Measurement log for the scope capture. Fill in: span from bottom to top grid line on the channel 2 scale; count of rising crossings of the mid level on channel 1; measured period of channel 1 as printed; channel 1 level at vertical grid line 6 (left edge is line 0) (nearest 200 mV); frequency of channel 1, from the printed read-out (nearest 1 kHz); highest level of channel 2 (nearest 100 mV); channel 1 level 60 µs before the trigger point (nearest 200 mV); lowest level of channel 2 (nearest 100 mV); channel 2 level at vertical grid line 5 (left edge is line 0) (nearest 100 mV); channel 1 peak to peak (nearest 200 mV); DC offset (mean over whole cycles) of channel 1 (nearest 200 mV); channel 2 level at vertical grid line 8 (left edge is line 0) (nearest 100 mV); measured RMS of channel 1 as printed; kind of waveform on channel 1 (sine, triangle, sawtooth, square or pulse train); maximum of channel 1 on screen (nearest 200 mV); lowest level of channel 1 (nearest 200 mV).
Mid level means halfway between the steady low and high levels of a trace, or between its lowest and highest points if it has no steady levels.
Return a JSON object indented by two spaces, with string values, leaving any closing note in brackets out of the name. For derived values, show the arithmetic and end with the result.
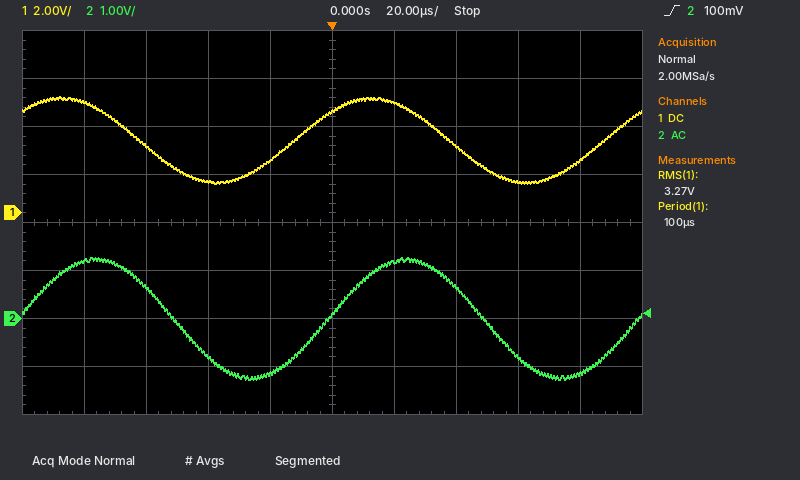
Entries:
{
  "span from bottom to top grid line on the channel 2 scale": "8 V",
  "count of rising crossings of the mid level on channel 1": "2",
  "measured period of channel 1 as printed": "100 µs",
  "channel 1 level at vertical grid line 6 (left edge is line 0)": "4.6 V",
  "frequency of channel 1, from the printed read-out": "1 / 100 µs ≈ 10 kHz",
  "highest level of channel 2": "1.3 V",
  "channel 1 level 60 µs before the trigger point": "2.8 V",
  "lowest level of channel 2": "-1.3 V",
  "channel 2 level at vertical grid line 5 (left edge is line 0)": "100 mV",
  "channel 1 peak to peak": "4.8 V − (1.2 V) = 3.6 V",
  "DC offset (mean over whole cycles) of channel 1": "(4.8 V + (1.2 V)) / 2 ≈ 3.0 V",
  "channel 2 level at vertical grid line 8 (left edge is line 0)": "-800 mV",
  "measured RMS of channel 1 as printed": "3.27 V",
  "kind of waveform on channel 1": "sine",
  "maximum of channel 1 on screen": "4.8 V",
  "lowest level of channel 1": "1.2 V"
}
